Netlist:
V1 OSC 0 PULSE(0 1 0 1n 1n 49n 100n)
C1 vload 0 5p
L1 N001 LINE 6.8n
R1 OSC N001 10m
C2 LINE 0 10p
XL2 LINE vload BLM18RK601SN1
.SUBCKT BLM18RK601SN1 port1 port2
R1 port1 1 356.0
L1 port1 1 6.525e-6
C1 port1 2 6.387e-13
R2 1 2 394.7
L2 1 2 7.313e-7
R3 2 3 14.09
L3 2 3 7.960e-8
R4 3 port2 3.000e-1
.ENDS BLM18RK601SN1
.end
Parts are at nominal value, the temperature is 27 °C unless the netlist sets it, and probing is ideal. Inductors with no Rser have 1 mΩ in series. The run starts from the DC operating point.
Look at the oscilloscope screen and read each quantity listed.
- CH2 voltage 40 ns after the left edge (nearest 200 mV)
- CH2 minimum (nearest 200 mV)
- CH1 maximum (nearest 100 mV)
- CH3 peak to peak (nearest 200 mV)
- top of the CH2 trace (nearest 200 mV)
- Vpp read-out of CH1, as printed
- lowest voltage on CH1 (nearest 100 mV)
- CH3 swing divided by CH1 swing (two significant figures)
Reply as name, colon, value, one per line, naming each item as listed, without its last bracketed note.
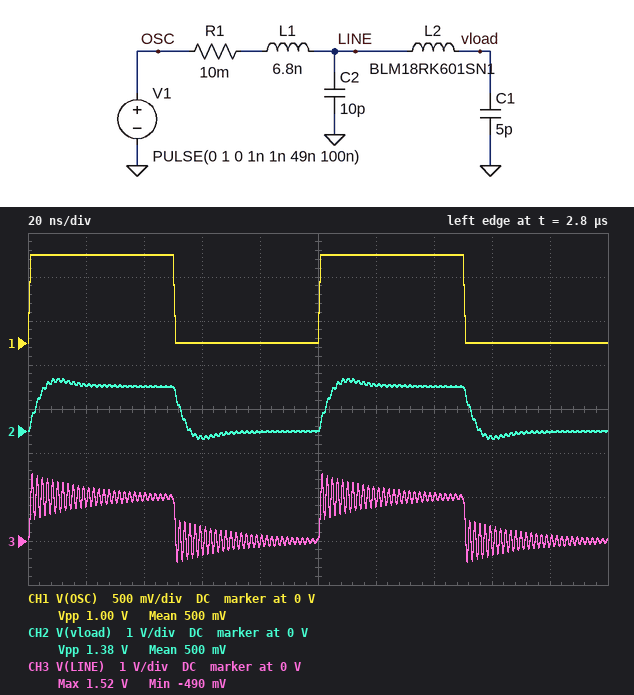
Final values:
CH2 voltage 40 ns after the left edge: 1.0 V
CH2 minimum: -200 mV
CH1 maximum: 1.0 V
CH3 peak to peak: 2.0 V
top of the CH2 trace: 1.2 V
Vpp read-out of CH1, as printed: 1.00 V
lowest voltage on CH1: 0 V
CH3 swing divided by CH1 swing: 2.0
